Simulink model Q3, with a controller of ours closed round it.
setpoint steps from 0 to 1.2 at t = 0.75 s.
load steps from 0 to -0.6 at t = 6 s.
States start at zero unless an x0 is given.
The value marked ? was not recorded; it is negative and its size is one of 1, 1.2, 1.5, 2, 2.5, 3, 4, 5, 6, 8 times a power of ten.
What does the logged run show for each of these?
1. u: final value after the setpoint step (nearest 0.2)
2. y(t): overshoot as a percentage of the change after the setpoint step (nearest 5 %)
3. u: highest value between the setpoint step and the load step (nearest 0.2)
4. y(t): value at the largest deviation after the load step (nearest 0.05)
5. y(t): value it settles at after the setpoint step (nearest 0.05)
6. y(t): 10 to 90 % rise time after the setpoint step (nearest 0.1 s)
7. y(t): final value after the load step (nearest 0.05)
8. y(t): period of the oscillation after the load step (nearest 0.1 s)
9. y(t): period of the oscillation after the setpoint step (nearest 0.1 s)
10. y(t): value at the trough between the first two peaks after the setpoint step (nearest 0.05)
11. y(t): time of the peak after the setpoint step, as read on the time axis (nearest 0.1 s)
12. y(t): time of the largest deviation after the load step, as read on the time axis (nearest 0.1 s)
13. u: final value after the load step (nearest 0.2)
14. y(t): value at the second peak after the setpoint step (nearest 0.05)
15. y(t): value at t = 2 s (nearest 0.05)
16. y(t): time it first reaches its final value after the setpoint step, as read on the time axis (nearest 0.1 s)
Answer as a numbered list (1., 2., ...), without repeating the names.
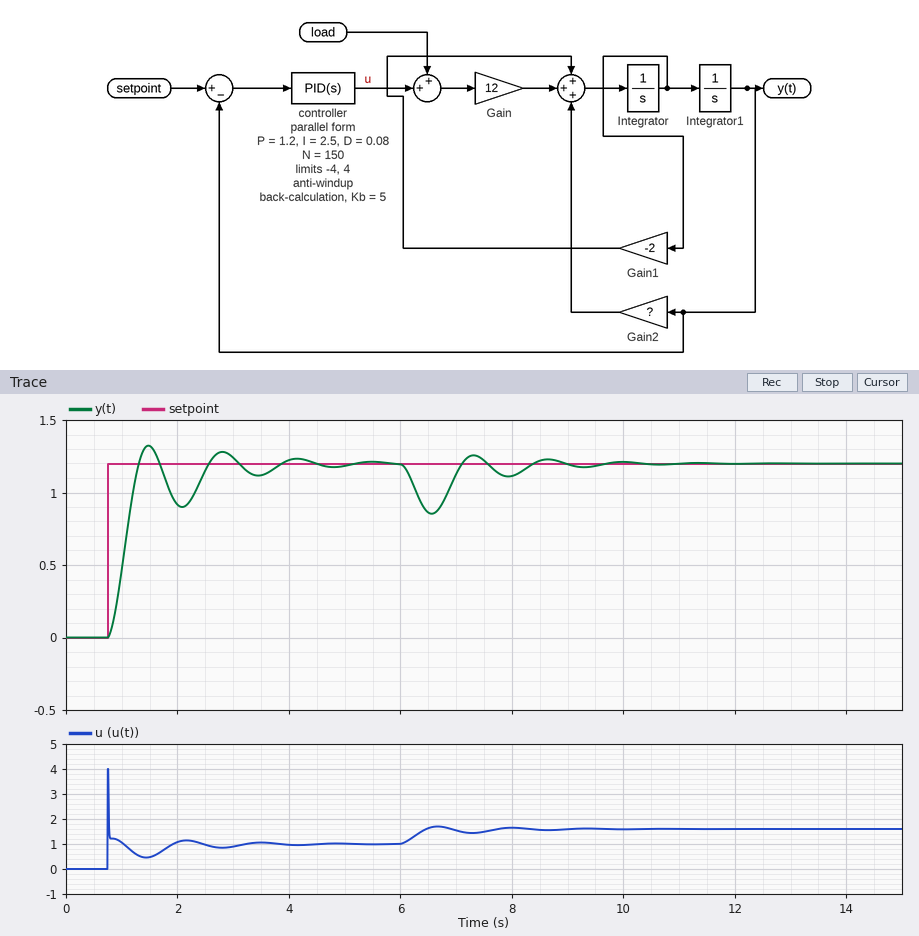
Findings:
1. 1.0
2. 10 %
3. 4.0
4. 0.85
5. 1.20
6. 0.4 s
7. 1.20
8. 1.4 s
9. 1.3 s
10. 0.90
11. 1.5 s
12. 6.6 s
13. 1.6
14. 1.30
15. 0.90
16. 1.3 s
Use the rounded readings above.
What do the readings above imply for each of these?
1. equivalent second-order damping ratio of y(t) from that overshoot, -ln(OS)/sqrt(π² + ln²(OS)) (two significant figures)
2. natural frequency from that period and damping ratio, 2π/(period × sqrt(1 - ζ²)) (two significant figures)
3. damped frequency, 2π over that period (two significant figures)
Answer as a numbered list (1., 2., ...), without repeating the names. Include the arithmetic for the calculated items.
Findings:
1. ln(0.1) = -2.303; 2.303 / sqrt(9.870 + 5.302) = 0.59
2. 2π / (1.3 × sqrt(1 - 0.59²)) = 6.0 rad/s
3. 2π / 1.3 = 4.8 rad/s
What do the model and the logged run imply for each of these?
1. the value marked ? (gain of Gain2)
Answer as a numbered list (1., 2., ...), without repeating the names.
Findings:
1. -10
